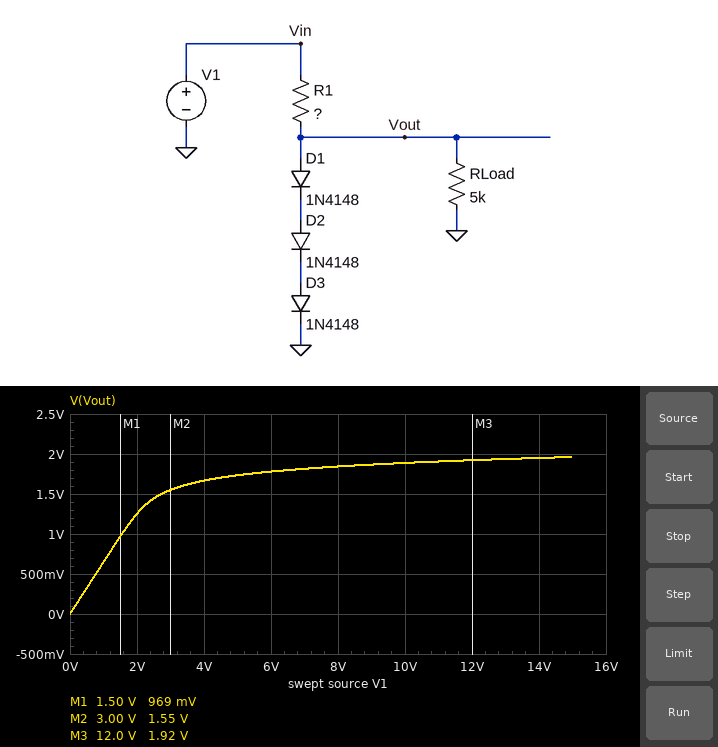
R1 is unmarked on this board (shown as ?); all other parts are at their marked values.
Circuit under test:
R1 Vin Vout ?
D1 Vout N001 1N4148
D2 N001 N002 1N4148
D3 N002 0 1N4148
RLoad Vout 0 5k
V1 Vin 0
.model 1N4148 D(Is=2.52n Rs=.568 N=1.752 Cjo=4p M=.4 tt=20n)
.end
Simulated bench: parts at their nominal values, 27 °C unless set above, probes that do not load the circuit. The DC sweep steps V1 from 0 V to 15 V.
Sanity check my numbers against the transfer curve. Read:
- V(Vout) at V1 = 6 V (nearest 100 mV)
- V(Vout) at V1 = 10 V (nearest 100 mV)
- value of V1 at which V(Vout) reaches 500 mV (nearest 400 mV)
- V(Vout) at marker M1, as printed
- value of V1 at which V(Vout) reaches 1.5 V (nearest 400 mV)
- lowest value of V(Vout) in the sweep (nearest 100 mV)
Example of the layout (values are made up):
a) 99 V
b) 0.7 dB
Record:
a) 1.8 V
b) 1.9 V
c) 800 mV
d) 969 mV
e) 2.8 V
f) 0 V
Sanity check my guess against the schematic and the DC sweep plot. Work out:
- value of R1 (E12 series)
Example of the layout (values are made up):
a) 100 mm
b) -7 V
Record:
a) 2.7 kΩ
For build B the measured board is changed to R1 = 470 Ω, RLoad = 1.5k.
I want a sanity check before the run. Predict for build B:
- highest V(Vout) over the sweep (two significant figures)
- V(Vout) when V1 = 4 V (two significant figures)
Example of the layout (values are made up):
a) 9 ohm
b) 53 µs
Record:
a) 2.2 V
b) 1.9 V
